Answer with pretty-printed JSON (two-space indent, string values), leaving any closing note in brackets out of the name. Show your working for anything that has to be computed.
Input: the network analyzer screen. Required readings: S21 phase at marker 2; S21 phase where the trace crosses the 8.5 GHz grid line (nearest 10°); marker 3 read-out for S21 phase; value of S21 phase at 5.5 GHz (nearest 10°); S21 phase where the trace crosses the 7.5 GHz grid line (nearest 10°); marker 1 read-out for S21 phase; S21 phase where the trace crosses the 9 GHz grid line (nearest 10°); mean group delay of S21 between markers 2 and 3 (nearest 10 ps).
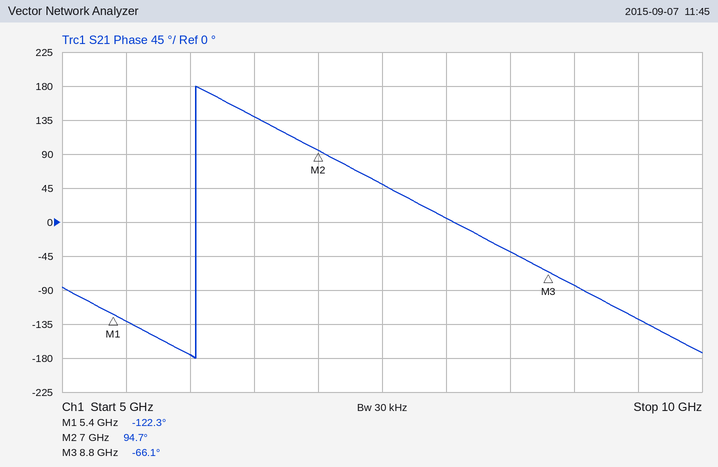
{
  "S21 phase at marker 2": "94.7°",
  "S21 phase where the trace crosses the 8.5 GHz grid line": "-40°",
  "marker 3 read-out for S21 phase": "-66.1°",
  "value of S21 phase at 5.5 GHz": "-130°",
  "S21 phase where the trace crosses the 7.5 GHz grid line": "50°",
  "marker 1 read-out for S21 phase": "-122.3°",
  "S21 phase where the trace crosses the 9 GHz grid line": "-80°",
  "mean group delay of S21 between markers 2 and 3": "−(-66.1° − (94.7°))/(360° × 1.8 GHz) ≈ 248 ps, so 250 ps to the nearest 10 ps"
}
